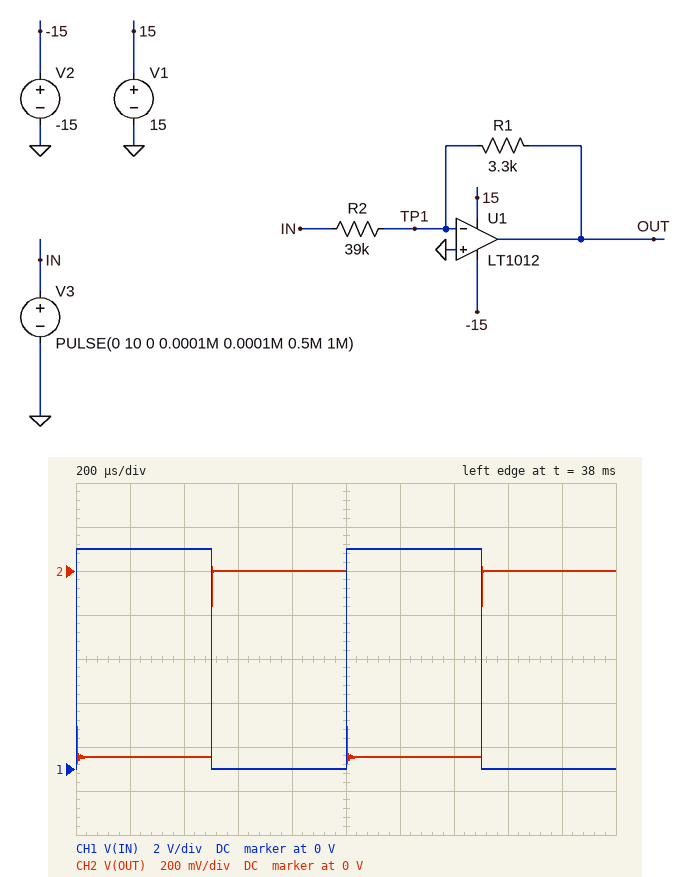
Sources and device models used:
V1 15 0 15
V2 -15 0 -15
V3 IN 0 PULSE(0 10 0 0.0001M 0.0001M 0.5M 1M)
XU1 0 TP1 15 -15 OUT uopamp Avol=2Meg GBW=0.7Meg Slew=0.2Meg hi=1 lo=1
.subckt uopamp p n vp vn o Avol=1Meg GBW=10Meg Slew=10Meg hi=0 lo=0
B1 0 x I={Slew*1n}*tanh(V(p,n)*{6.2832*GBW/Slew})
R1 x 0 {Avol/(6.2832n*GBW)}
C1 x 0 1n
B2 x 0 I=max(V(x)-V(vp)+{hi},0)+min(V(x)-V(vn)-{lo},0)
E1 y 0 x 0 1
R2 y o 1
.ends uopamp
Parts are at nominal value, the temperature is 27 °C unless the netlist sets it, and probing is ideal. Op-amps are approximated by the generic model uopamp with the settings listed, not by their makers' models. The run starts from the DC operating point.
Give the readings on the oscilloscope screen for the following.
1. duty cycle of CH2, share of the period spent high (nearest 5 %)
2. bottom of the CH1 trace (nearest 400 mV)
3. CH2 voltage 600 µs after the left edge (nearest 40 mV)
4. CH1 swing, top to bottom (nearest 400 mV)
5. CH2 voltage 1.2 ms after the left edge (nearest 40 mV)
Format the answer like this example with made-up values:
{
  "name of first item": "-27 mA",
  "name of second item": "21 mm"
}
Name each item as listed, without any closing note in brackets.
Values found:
{
  "duty cycle of CH2, share of the period spent high": "50 %",
  "bottom of the CH1 trace": "0 V",
  "CH2 voltage 600 µs after the left edge": "0 V",
  "CH1 swing, top to bottom": "10.0 V",
  "CH2 voltage 1.2 ms after the left edge": "-840 mV"
}
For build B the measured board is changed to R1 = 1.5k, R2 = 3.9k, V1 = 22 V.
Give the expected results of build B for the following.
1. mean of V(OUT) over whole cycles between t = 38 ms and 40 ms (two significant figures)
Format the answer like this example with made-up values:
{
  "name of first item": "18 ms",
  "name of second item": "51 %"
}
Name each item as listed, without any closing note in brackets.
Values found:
{
  "mean of V(OUT) over whole cycles between t = 38 ms and 40 ms": "-1.9 V"
}
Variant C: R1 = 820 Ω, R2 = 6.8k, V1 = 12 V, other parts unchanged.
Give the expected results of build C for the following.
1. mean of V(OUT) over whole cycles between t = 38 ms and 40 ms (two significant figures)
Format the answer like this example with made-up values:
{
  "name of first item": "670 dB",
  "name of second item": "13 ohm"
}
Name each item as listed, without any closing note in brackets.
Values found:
{
  "mean of V(OUT) over whole cycles between t = 38 ms and 40 ms": "-600 mV"
}
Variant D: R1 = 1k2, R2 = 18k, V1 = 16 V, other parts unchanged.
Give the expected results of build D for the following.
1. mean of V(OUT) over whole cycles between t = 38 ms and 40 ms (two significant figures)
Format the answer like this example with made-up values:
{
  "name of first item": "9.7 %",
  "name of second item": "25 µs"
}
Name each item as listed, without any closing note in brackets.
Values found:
{
  "mean of V(OUT) over whole cycles between t = 38 ms and 40 ms": "-330 mV"
}
